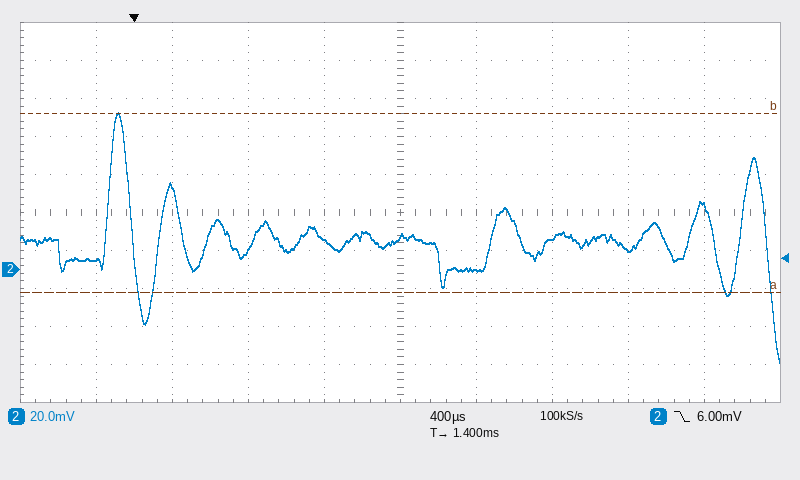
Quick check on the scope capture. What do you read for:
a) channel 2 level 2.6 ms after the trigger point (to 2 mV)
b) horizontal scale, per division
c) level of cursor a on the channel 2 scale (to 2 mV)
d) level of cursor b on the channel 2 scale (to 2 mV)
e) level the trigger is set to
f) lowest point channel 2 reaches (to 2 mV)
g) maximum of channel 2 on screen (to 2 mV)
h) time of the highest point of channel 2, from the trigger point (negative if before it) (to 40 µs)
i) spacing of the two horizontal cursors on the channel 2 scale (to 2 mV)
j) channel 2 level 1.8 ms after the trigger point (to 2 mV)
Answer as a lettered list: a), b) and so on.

a) 10 mV
b) 400 µs
c) -12 mV
d) 82 mV
e) 6.00 mV
f) -48 mV
g) 82 mV
h) -80 µs
i) 94 mV
j) 0 mV
